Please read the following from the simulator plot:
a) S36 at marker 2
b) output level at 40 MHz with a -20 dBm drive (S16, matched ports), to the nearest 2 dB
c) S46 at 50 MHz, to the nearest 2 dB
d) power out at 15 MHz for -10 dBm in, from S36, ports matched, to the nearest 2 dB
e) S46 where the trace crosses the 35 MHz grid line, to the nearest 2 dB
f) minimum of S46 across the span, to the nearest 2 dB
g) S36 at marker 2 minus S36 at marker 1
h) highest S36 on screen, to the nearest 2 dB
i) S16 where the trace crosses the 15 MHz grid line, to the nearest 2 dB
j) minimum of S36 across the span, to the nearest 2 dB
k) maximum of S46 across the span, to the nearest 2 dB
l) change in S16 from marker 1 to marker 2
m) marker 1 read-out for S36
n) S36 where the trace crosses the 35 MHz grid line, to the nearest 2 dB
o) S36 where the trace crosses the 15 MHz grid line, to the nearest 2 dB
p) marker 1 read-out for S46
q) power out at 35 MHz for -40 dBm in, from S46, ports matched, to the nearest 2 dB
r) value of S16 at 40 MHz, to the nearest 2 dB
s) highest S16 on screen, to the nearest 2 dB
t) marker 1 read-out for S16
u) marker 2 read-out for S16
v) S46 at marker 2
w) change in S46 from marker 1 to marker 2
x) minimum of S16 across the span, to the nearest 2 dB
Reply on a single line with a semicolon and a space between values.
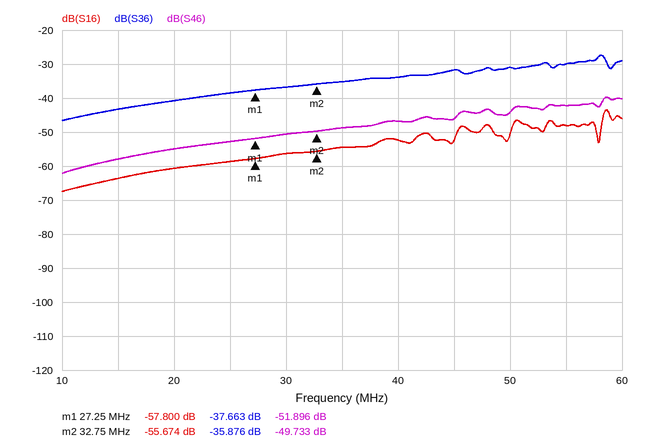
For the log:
-35.876 dB; -72 dBm; -44 dB; -54 dBm; -48 dB; -62 dB; 1.787 dB; -28 dB; -64 dB; -46 dB; -40 dB; 2.126 dB; -37.663 dB; -36 dB; -44 dB; -51.896 dB; -88 dBm; -52 dB; -44 dB; -57.800 dB; -55.674 dB; -49.733 dB; 2.163 dB; -68 dB
